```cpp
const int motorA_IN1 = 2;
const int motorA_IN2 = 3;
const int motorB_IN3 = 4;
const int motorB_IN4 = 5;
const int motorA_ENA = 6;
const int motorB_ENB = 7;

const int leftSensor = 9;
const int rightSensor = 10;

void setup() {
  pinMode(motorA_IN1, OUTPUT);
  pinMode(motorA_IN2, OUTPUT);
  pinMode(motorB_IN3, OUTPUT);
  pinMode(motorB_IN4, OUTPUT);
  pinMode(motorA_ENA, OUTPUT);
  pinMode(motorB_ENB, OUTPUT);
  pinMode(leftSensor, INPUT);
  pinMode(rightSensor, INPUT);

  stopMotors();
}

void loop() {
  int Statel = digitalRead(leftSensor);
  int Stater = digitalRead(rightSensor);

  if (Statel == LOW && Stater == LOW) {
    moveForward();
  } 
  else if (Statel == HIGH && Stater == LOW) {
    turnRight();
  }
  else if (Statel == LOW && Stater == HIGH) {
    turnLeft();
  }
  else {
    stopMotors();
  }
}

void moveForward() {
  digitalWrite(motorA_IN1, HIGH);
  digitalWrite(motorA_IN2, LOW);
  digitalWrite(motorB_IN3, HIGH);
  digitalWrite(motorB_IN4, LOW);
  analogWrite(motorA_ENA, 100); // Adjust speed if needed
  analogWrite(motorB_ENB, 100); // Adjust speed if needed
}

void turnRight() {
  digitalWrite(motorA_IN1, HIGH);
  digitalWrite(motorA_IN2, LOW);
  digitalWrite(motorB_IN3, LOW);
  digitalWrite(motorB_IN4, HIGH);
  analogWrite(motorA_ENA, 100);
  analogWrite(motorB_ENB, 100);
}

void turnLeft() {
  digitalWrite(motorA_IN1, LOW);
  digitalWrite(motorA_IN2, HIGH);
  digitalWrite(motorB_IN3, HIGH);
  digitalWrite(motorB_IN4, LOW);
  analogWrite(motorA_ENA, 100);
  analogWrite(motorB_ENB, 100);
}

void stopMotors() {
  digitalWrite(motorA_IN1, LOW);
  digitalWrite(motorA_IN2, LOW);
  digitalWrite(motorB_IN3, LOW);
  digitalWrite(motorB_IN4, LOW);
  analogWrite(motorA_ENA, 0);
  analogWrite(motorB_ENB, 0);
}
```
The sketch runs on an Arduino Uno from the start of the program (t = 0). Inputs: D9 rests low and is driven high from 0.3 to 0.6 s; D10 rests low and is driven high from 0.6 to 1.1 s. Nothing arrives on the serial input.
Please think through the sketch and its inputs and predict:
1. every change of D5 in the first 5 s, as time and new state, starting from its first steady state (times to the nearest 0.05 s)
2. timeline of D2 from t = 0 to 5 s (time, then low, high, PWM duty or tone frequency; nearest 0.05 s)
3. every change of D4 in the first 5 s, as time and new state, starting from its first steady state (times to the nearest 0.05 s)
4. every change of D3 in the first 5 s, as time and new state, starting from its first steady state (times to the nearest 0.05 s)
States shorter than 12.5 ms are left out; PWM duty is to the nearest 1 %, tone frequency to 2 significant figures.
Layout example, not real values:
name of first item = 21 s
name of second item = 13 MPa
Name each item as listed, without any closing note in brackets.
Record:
every change of D5 in the first 5 s, as time and new state, starting from its first steady state = 0 s low; 0.3 s high; 0.6 s low
timeline of D2 from t = 0 to 5 s = 0 s high; 0.6 s low; 1.1 s high
every change of D4 in the first 5 s, as time and new state, starting from its first steady state = 0 s high; 0.3 s low; 0.6 s high
every change of D3 in the first 5 s, as time and new state, starting from its first steady state = 0 s low; 0.6 s high; 1.1 s low
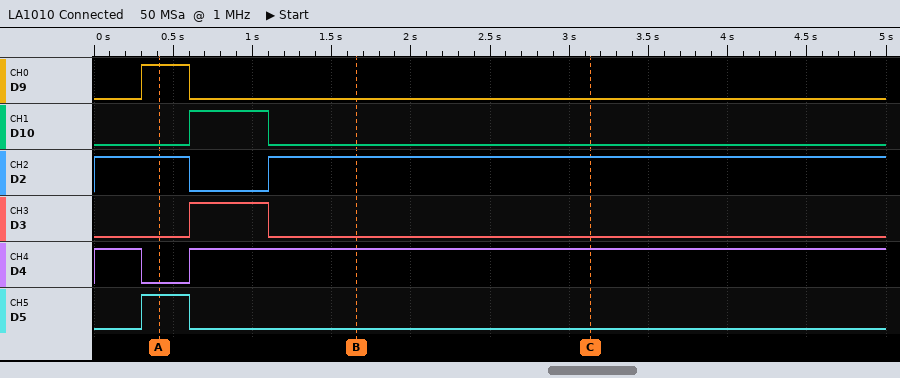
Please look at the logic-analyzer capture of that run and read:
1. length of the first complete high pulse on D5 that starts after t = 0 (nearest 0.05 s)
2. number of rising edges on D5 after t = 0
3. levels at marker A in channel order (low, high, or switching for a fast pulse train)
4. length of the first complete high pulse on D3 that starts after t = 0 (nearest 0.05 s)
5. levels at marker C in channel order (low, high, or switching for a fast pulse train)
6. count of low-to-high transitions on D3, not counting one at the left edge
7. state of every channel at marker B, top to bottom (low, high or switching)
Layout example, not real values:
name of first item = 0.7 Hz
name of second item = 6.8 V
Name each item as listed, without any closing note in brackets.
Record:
length of the first complete high pulse on D5 that starts after t = 0 = 0.30 s
number of rising edges on D5 after t = 0 = 1
levels at marker A in channel order = D9 high, D10 low, D2 high, D3 low, D4 low, D5 high
length of the first complete high pulse on D3 that starts after t = 0 = 0.50 s
levels at marker C in channel order = D9 low, D10 low, D2 high, D3 low, D4 high, D5 low
count of low-to-high transitions on D3, not counting one at the left edge = 1
state of every channel at marker B, top to bottom = D9 low, D10 low, D2 high, D3 low, D4 high, D5 low
